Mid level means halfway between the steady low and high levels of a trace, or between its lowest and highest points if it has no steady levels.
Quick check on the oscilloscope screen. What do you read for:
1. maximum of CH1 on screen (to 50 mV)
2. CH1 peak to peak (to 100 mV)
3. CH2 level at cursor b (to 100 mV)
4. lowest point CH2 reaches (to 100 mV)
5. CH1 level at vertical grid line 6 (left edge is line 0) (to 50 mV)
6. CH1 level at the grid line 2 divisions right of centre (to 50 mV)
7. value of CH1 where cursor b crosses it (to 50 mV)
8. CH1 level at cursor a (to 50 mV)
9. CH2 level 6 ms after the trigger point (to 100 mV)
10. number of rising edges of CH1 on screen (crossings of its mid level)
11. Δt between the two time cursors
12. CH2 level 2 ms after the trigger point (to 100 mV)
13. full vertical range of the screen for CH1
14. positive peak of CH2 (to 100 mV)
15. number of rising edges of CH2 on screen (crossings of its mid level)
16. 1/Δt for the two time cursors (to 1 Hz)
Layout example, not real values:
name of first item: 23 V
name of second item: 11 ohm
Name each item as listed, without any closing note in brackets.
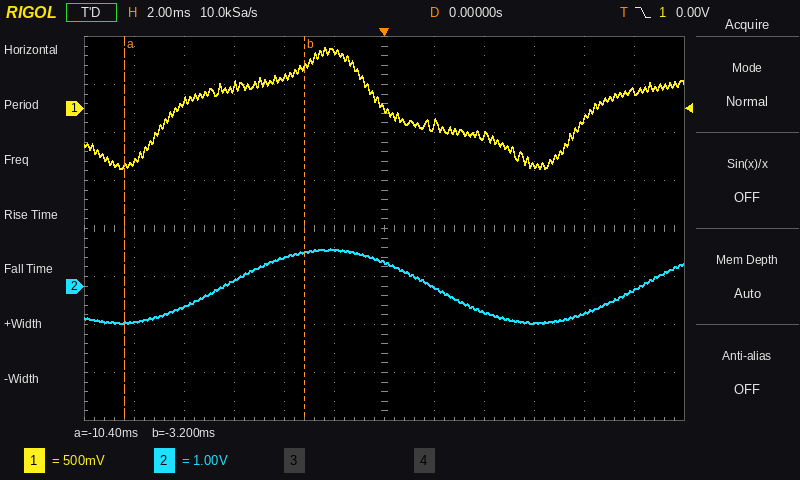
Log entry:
maximum of CH1 on screen: 650 mV
CH1 peak to peak: 1.30 V
CH2 level at cursor b: 700 mV
lowest point CH2 reaches: -800 mV
CH1 level at vertical grid line 6 (left edge is line 0): 0 mV
CH1 level at the grid line 2 divisions right of centre: -300 mV
value of CH1 where cursor b crosses it: 450 mV
CH1 level at cursor a: -600 mV
CH2 level 6 ms after the trigger point: -800 mV
number of rising edges of CH1 on screen: 2
Δt between the two time cursors: 7.2 ms
CH2 level 2 ms after the trigger point: 0.0 V
full vertical range of the screen for CH1: 4 V
positive peak of CH2: 800 mV
number of rising edges of CH2 on screen: 2
1/Δt for the two time cursors: 139 Hz
